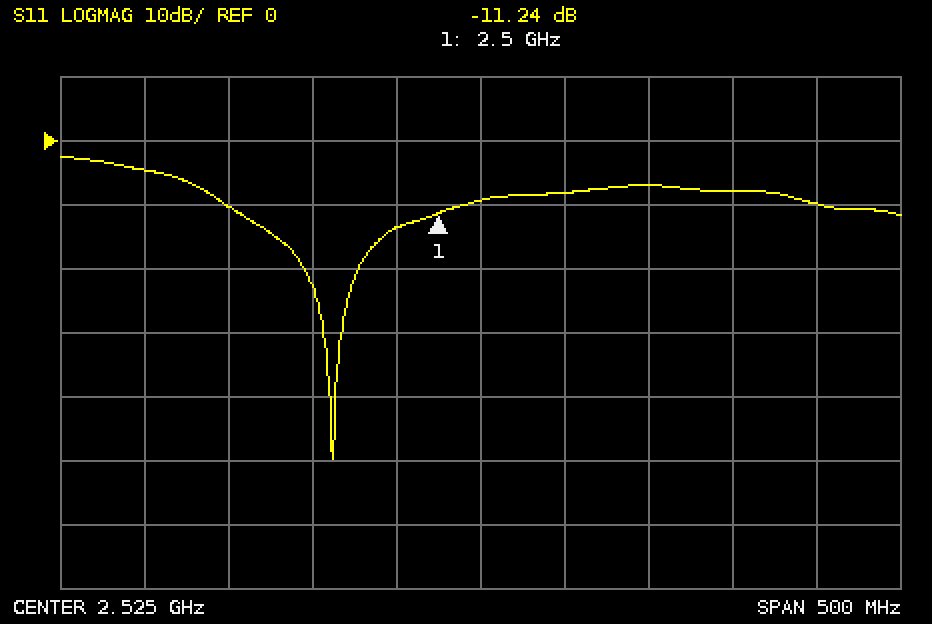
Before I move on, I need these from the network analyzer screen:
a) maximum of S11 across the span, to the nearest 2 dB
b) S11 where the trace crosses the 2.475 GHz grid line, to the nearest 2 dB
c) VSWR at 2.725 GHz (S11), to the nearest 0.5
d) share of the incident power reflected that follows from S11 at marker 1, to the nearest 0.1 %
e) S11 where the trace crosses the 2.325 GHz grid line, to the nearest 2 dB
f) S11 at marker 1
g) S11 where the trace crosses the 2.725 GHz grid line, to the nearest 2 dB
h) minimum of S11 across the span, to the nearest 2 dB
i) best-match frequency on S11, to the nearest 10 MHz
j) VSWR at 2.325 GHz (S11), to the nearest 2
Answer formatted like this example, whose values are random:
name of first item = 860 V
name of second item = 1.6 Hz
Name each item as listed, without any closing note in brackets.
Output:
maximum of S11 across the span, to the nearest 2 dB = -2 dB
S11 where the trace crosses the 2.475 GHz grid line, to the nearest 2 dB = -14 dB
VSWR at 2.725 GHz (S11), to the nearest 0.5 = 2.0
share of the incident power reflected that follows from S11 at marker 1, to the nearest 0.1 % = 7.5 %
S11 where the trace crosses the 2.325 GHz grid line, to the nearest 2 dB = -4 dB
S11 at marker 1 = -11.24 dB
S11 where the trace crosses the 2.725 GHz grid line, to the nearest 2 dB = -10 dB
minimum of S11 across the span, to the nearest 2 dB = -50 dB
best-match frequency on S11, to the nearest 10 MHz = 2.44 GHz
VSWR at 2.325 GHz (S11), to the nearest 2 = 4
